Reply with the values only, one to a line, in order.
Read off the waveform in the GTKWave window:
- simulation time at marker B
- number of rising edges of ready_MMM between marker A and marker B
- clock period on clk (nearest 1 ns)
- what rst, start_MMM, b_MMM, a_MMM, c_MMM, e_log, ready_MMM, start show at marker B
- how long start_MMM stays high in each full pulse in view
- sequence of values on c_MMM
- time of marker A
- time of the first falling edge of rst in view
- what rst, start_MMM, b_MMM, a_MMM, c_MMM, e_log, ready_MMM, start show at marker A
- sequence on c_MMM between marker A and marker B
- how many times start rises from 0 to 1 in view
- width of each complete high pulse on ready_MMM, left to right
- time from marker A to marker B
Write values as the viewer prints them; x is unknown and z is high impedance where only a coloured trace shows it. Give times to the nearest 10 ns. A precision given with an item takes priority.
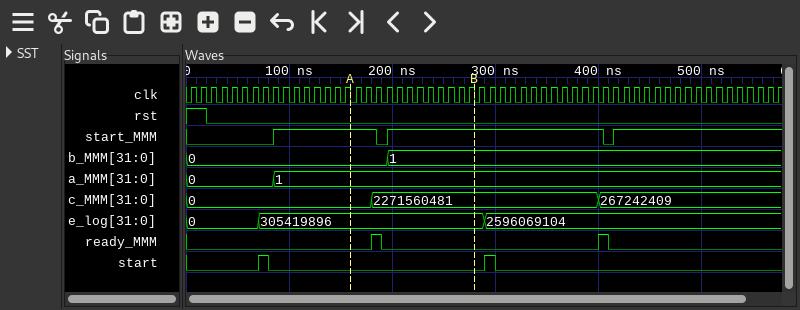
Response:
280 ns
1
10 ns
rst=0, start_MMM=1, b_MMM=1, a_MMM=1, c_MMM=2271560481, e_log=305419896, ready_MMM=0, start=0
100 ns, 210 ns
0, 2271560481, 267242409
160 ns
20 ns
rst=0, start_MMM=1, b_MMM=0, a_MMM=1, c_MMM=0, e_log=305419896, ready_MMM=0, start=0
0, 2271560481
2
10 ns, 10 ns
120 ns
